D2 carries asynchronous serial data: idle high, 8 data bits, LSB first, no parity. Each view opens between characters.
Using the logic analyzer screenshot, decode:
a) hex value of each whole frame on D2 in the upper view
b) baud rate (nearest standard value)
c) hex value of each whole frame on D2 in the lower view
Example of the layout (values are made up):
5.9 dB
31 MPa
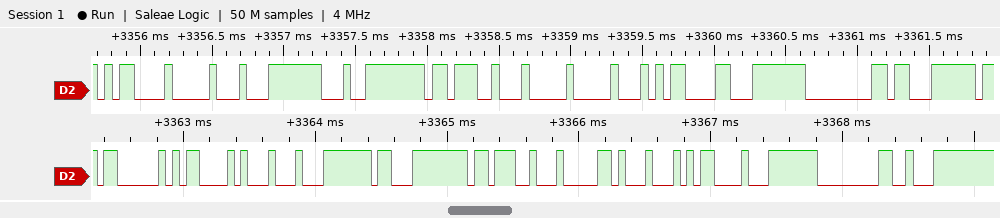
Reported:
0D, 10, FC, E4, 3B, 04, 10, 0D, FC, 00, E3
19200 baud
03, 0D, 11, FC, E3, 3B, 04, 11, 0D, FC, 00, E2
